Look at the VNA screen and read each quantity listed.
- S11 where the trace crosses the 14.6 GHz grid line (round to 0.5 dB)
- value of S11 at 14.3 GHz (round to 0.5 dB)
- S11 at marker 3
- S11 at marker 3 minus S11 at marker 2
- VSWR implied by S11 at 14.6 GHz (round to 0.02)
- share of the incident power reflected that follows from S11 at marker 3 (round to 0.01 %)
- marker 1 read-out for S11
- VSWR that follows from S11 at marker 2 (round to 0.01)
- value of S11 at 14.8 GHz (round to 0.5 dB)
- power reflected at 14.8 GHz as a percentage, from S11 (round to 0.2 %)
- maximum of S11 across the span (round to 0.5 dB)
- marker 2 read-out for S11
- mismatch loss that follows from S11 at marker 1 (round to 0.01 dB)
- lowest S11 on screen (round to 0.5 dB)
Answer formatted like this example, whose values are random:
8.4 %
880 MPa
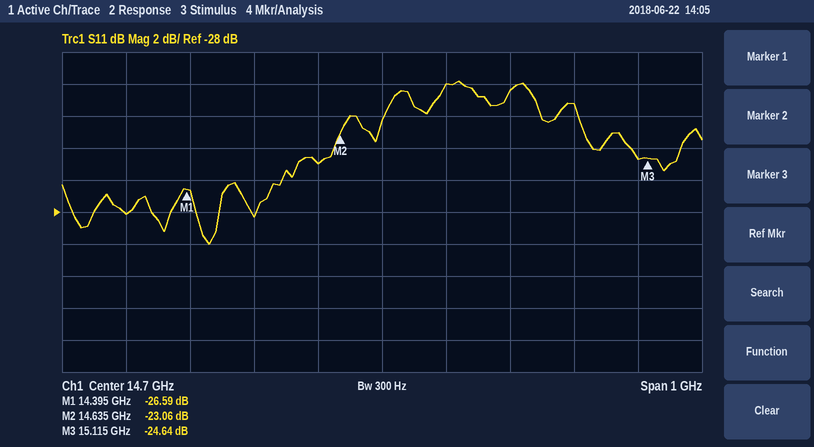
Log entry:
-25.0 dB
-28.0 dB
-24.64 dB
-1.58 dB
1.12
0.34 %
-26.59 dB
1.15
-20.0 dB
1.0 %
-20.0 dB
-23.06 dB
0.01 dB
-30.0 dB
